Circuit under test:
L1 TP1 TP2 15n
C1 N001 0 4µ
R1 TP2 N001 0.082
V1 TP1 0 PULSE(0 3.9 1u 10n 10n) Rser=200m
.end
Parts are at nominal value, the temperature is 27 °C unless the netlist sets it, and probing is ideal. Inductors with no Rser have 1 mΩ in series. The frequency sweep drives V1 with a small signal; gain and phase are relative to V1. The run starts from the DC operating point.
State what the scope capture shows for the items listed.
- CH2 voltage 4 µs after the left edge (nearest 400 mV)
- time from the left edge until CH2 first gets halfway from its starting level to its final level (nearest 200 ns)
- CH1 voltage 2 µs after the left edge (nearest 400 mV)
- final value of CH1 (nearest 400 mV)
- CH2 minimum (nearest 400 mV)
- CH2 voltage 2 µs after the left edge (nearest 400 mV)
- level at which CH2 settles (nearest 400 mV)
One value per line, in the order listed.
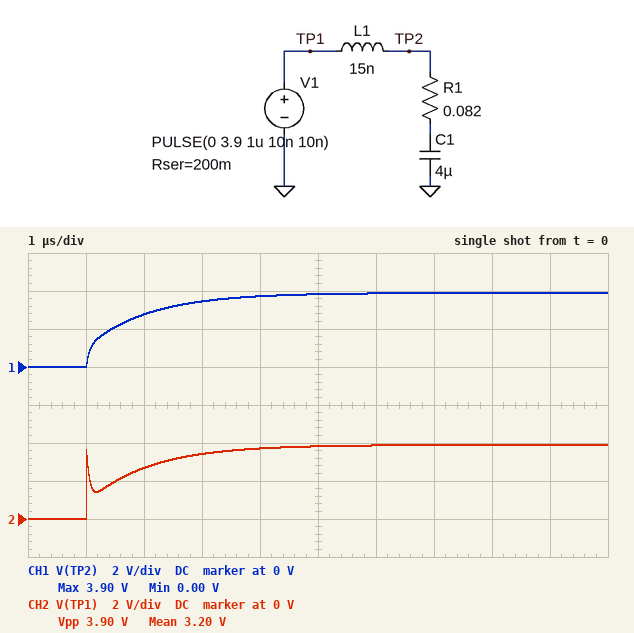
3.6 V
1.0 µs
2.8 V
4.0 V
0 V
2.8 V
4.0 V
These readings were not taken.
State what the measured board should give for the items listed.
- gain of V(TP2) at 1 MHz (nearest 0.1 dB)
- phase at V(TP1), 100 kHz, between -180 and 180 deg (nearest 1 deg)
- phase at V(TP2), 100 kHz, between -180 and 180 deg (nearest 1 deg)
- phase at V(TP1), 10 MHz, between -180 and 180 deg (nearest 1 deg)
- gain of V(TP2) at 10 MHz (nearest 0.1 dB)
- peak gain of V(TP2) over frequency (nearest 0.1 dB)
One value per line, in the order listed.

-10.0 dB
-24 deg
-24 deg
12 deg
-21.5 dB
0 dB
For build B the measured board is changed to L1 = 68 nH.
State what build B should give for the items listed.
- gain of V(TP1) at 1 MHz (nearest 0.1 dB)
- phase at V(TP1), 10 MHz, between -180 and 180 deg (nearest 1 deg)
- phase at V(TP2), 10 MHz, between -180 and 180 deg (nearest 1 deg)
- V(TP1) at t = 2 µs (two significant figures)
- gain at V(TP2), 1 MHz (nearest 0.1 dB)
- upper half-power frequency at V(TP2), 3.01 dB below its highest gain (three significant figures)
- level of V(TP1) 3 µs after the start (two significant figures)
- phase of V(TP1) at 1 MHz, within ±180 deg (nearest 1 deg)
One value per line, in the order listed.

-1.7 dB
3 deg
-89 deg
2.3 V
-14.4 dB
199 kHz
3.4 V
24 deg
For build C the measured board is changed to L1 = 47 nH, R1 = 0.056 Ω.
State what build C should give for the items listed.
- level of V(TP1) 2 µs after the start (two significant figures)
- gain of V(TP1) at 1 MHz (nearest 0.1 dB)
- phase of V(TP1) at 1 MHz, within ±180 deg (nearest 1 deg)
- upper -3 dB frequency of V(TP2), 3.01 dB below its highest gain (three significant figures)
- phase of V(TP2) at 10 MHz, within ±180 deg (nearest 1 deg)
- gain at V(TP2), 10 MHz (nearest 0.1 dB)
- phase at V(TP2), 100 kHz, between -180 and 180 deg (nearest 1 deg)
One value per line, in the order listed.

2.4 V
-2.8 dB
33 deg
200 kHz
-89 deg
-34.4 dB
-27 deg
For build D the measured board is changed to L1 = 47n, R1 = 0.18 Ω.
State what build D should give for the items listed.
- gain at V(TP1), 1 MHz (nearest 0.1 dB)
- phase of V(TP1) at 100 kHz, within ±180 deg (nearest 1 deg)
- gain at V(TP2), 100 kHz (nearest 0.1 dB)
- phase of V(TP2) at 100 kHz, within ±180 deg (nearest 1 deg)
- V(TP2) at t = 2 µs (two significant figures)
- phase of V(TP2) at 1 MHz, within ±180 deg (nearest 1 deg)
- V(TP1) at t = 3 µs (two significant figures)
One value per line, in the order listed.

-3.3 dB
-20 deg
-1.7 dB
-22 deg
2.9 V
-46 deg
3.3 V
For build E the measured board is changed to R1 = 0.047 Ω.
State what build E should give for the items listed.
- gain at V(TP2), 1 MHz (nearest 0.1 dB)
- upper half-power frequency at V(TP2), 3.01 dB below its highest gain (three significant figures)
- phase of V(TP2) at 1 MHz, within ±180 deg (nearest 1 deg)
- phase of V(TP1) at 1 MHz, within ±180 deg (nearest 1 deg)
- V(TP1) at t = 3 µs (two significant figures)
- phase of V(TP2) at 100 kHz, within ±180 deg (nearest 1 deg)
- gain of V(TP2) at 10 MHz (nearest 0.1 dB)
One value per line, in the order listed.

-12.3 dB
178 kHz
-53 deg
36 deg
3.5 V
-26 deg
-26.3 dB
